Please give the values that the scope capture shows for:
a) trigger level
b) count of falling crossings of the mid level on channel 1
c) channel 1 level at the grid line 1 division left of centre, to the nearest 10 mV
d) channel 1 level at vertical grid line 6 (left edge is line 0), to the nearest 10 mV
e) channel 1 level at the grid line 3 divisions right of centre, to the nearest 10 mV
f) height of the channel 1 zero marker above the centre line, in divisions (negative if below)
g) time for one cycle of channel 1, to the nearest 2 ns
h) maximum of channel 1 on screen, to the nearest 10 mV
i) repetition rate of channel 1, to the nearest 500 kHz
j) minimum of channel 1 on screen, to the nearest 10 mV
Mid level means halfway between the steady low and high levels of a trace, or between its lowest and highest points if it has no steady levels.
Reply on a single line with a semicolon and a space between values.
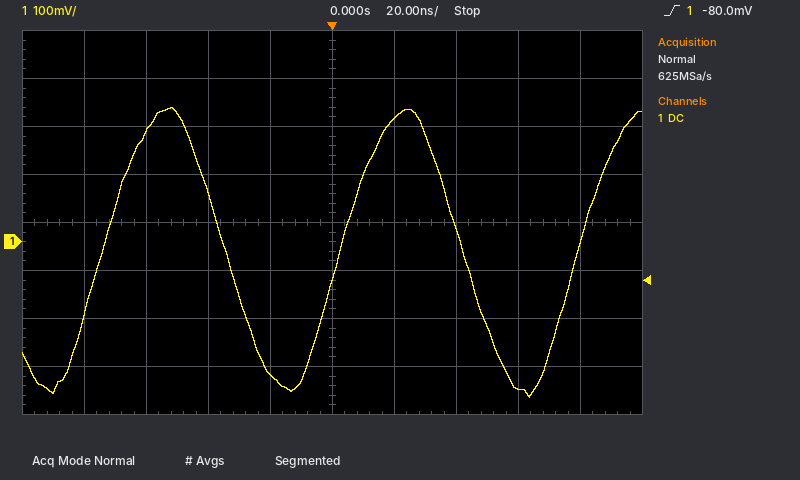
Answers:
-80.0 mV; 2; -280 mV; 260 mV; -310 mV; -0.4 div; 76 ns; 280 mV; 13.0 MHz; -320 mV
